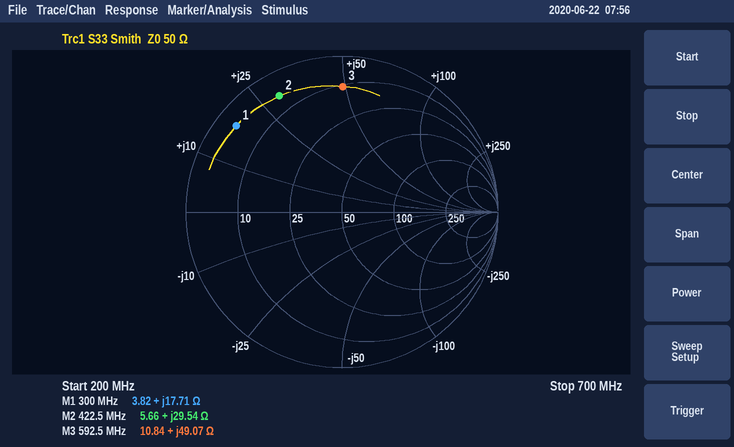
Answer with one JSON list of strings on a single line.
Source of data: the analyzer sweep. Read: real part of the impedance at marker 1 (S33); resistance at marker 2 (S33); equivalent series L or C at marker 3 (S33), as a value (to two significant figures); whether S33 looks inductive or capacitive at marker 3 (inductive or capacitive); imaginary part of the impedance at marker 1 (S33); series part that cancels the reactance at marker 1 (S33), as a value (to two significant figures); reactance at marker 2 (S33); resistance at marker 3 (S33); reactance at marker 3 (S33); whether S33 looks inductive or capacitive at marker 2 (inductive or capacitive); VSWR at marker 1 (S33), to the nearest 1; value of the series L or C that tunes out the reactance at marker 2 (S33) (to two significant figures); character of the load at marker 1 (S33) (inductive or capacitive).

["3.82 Ω", "5.66 Ω", "13 nH", "inductive", "+17.71 Ω", "30 pF", "+29.54 Ω", "10.84 Ω", "+49.07 Ω", "inductive", "15", "13 pF", "inductive"]
